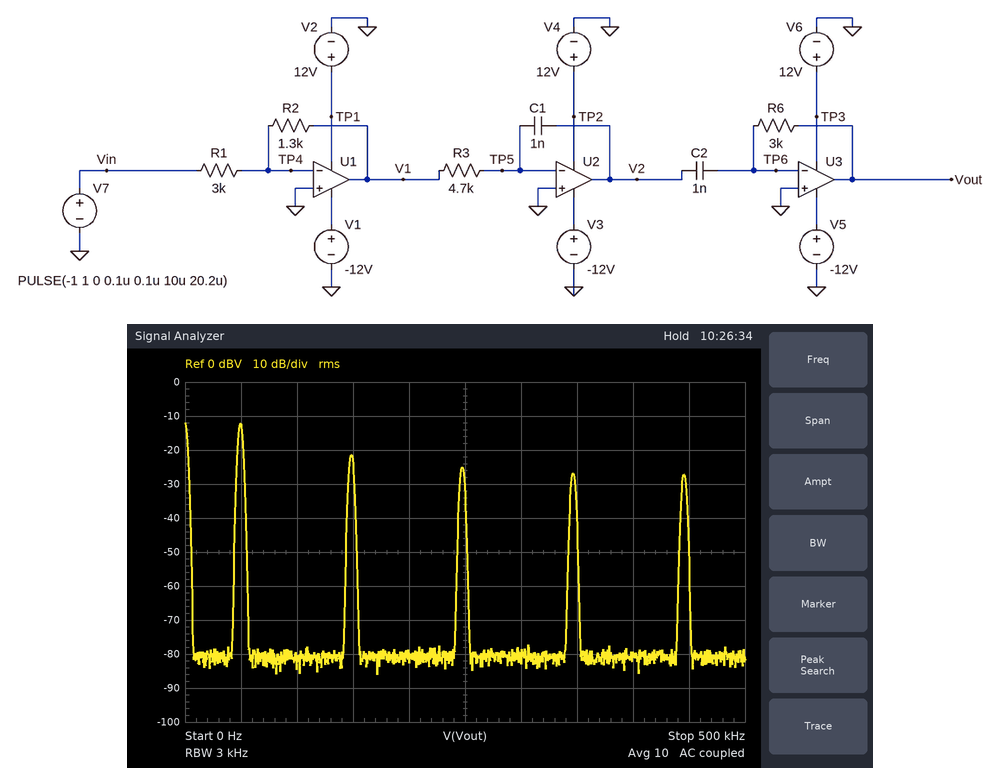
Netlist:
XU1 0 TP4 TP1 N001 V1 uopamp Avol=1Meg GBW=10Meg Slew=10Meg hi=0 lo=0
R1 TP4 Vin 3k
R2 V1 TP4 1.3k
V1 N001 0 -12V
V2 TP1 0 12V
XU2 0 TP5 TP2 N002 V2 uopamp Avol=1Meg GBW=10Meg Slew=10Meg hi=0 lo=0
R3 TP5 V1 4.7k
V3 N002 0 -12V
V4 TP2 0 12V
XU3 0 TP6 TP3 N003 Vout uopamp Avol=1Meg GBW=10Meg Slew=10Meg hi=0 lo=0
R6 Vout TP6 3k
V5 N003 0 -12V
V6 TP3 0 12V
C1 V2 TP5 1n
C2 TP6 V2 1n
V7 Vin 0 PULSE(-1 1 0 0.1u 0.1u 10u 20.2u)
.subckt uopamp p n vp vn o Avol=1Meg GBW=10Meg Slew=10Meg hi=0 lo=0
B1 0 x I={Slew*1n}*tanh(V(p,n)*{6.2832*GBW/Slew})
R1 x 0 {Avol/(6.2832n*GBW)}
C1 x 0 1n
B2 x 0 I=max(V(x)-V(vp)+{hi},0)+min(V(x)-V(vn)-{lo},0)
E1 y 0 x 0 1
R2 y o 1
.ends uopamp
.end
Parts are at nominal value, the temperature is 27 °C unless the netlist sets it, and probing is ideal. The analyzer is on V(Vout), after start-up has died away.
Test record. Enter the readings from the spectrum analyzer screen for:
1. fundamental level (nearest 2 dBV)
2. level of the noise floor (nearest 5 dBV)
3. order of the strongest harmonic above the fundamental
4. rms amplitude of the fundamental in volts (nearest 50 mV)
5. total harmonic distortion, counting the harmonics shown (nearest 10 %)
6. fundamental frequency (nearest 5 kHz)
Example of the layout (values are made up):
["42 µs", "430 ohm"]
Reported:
["-12 dBV", "-80 dBV", "3", "250 mV", "50 %", "50 kHz"]
